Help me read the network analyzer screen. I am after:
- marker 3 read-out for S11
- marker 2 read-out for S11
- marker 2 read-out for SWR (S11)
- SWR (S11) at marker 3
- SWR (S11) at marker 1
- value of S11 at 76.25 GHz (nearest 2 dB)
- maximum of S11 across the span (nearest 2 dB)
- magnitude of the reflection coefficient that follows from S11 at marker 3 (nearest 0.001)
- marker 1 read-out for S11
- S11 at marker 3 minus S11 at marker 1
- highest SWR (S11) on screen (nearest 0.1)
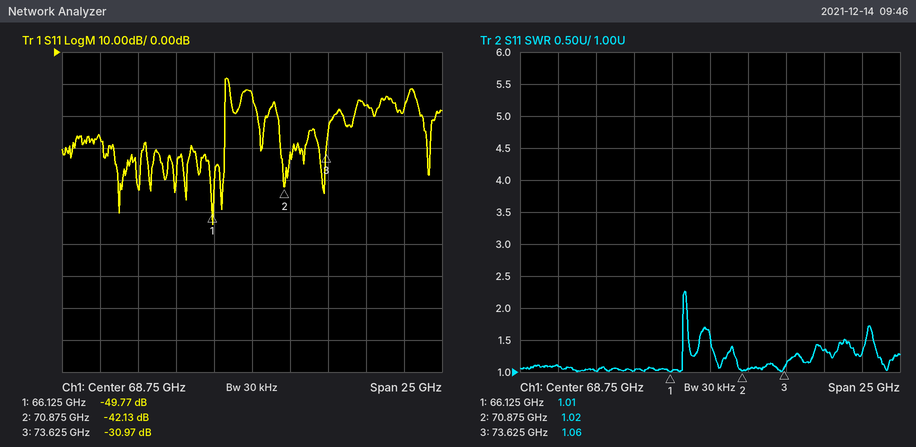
-30.97 dB
-42.13 dB
1.02
1.06
1.01
-16 dB
-8 dB
0.028
-49.77 dB
18.80 dB
2.3
